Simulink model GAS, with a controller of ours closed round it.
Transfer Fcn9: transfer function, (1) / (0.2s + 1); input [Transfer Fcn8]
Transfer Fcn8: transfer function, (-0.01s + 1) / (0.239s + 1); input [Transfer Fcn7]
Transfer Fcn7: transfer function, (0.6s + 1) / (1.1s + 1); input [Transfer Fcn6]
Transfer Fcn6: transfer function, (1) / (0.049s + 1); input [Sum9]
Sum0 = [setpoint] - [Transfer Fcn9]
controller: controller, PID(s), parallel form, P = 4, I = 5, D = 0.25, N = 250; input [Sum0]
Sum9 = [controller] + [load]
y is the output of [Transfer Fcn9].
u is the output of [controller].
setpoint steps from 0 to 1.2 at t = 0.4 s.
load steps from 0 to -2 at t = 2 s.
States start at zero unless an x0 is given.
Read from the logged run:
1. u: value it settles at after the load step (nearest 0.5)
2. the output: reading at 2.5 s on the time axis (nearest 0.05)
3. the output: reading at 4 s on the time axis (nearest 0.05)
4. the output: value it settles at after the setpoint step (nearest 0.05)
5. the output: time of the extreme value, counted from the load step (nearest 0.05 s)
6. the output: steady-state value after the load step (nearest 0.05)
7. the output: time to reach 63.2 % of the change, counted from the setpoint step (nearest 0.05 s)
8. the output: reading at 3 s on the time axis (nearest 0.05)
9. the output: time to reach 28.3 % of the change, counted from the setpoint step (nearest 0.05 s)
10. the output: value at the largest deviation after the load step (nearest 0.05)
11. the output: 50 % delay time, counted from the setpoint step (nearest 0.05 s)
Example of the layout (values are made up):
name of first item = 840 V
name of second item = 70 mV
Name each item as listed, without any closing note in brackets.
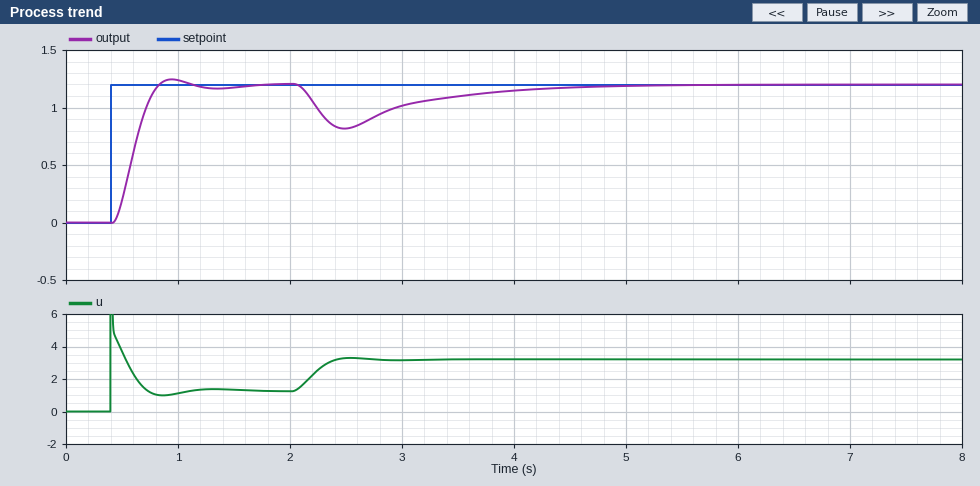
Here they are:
u: value it settles at after the load step = 3.0
the output: reading at 2.5 s on the time axis = 0.80
the output: reading at 4 s on the time axis = 1.15
the output: value it settles at after the setpoint step = 1.20
the output: time of the extreme value, counted from the load step = 0.50 s
the output: steady-state value after the load step = 1.20
the output: time to reach 63.2 % of the change, counted from the setpoint step = 0.25 s
the output: reading at 3 s on the time axis = 1.00
the output: time to reach 28.3 % of the change, counted from the setpoint step = 0.15 s
the output: value at the largest deviation after the load step = 0.80
the output: 50 % delay time, counted from the setpoint step = 0.20 s
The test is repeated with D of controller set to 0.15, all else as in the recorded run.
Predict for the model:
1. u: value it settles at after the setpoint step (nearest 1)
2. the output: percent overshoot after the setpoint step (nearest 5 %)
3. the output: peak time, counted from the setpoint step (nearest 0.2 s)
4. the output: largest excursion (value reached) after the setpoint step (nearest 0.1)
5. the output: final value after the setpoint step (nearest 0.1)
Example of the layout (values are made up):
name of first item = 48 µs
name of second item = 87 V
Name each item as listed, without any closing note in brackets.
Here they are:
u: value it settles at after the setpoint step = 1
the output: percent overshoot after the setpoint step = 10 %
the output: peak time, counted from the setpoint step = 0.6 s
the output: largest excursion (value reached) after the setpoint step = 1.3
the output: final value after the setpoint step = 1.2
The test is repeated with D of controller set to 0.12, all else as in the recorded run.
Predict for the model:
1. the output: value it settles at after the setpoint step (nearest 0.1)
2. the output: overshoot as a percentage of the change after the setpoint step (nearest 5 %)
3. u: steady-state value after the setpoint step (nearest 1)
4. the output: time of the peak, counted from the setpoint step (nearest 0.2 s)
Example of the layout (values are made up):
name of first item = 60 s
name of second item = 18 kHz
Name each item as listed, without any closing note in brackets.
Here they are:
the output: value it settles at after the setpoint step = 1.2
the output: overshoot as a percentage of the change after the setpoint step = 10 %
u: steady-state value after the setpoint step = 1
the output: time of the peak, counted from the setpoint step = 0.6 s
